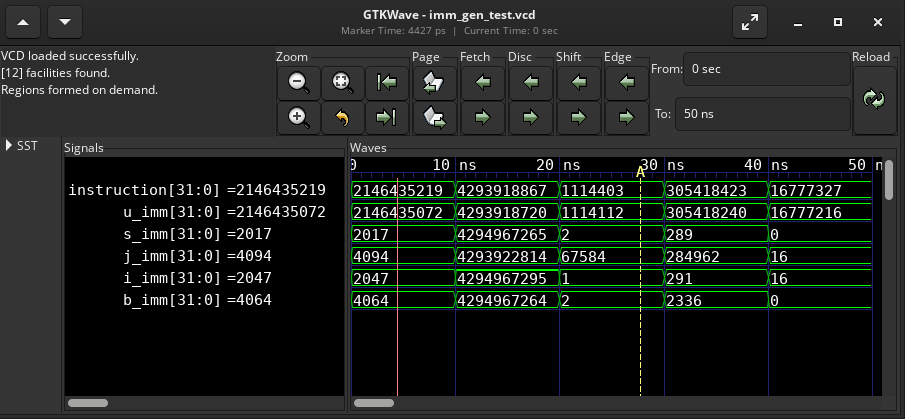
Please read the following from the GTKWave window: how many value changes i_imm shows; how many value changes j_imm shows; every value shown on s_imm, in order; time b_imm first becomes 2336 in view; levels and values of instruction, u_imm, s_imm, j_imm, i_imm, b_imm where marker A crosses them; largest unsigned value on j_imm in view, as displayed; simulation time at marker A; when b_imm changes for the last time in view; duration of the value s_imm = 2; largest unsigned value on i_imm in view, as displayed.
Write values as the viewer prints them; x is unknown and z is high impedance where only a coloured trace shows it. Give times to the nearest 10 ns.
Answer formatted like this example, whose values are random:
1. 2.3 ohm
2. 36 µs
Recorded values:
1. 4
2. 4
3. 2017, 4294967265, 2, 289, 0
4. 30 ns
5. instruction=1114403, u_imm=1114112, s_imm=2, j_imm=67584, i_imm=1, b_imm=2
6. 4293922814
7. 30 ns
8. 40 ns
9. 10 ns
10. 4294967295
